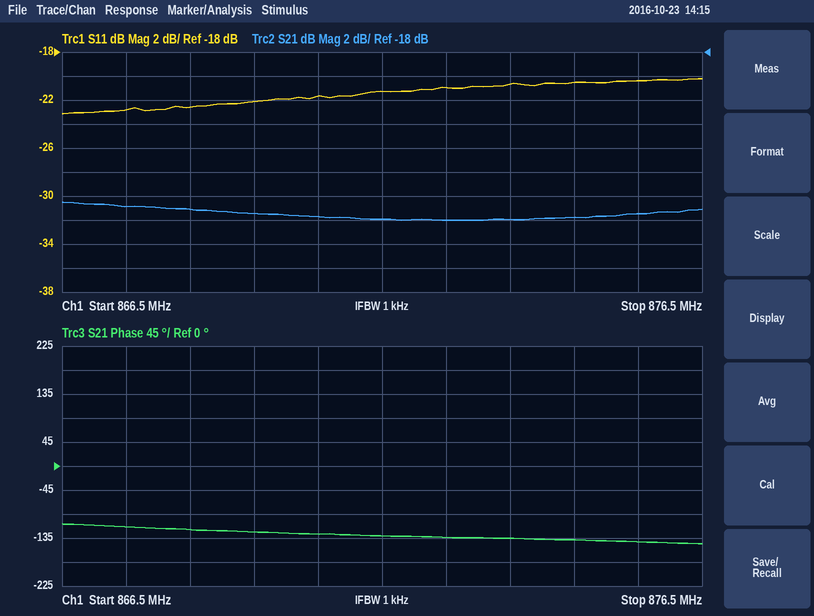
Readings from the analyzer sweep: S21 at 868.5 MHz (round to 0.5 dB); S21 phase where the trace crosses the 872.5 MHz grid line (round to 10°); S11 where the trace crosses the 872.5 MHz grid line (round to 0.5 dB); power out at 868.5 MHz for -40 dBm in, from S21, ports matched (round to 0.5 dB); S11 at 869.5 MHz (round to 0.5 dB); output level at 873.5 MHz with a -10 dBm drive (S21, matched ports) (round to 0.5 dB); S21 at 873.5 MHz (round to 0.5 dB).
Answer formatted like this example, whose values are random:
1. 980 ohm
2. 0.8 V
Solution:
1. -31.0 dB
2. -130°
3. -21.0 dB
4. -71.0 dBm
5. -22.0 dB
6. -42.0 dBm
7. -32.0 dB
